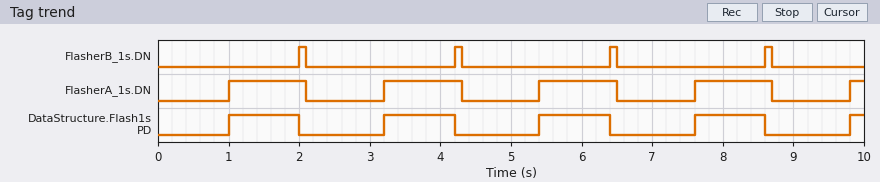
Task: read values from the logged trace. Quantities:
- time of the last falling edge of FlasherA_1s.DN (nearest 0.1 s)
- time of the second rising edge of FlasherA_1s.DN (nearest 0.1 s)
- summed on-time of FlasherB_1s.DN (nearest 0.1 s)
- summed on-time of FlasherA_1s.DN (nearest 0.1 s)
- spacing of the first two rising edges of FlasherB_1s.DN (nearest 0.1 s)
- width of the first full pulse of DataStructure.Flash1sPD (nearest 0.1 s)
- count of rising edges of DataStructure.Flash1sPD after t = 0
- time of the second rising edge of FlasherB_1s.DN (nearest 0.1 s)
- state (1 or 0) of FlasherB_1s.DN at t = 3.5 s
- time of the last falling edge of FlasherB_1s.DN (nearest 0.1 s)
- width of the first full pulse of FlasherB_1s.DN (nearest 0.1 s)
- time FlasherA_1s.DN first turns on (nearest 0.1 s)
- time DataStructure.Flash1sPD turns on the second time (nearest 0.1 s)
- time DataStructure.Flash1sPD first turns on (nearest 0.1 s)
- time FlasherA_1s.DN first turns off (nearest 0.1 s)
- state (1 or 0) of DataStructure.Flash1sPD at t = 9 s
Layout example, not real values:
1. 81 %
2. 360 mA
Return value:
1. 8.7 s
2. 3.2 s
3. 0.4 s
4. 4.6 s
5. 2.2 s
6. 1.0 s
7. 5
8. 4.2 s
9. 0
10. 8.7 s
11. 0.1 s
12. 1.0 s
13. 3.2 s
14. 1.0 s
15. 2.1 s
16. 0
